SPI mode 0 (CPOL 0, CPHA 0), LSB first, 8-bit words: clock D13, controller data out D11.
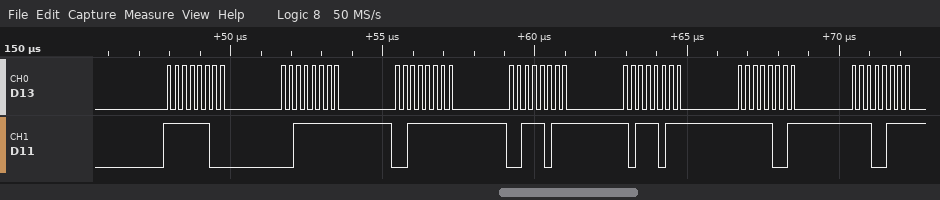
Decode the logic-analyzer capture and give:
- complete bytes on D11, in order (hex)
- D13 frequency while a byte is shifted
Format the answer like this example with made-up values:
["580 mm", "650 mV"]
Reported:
["0x3F 0xFC 0xFC 0xDC 0xDD 0x9F 0xE7", "4 MHz"]
